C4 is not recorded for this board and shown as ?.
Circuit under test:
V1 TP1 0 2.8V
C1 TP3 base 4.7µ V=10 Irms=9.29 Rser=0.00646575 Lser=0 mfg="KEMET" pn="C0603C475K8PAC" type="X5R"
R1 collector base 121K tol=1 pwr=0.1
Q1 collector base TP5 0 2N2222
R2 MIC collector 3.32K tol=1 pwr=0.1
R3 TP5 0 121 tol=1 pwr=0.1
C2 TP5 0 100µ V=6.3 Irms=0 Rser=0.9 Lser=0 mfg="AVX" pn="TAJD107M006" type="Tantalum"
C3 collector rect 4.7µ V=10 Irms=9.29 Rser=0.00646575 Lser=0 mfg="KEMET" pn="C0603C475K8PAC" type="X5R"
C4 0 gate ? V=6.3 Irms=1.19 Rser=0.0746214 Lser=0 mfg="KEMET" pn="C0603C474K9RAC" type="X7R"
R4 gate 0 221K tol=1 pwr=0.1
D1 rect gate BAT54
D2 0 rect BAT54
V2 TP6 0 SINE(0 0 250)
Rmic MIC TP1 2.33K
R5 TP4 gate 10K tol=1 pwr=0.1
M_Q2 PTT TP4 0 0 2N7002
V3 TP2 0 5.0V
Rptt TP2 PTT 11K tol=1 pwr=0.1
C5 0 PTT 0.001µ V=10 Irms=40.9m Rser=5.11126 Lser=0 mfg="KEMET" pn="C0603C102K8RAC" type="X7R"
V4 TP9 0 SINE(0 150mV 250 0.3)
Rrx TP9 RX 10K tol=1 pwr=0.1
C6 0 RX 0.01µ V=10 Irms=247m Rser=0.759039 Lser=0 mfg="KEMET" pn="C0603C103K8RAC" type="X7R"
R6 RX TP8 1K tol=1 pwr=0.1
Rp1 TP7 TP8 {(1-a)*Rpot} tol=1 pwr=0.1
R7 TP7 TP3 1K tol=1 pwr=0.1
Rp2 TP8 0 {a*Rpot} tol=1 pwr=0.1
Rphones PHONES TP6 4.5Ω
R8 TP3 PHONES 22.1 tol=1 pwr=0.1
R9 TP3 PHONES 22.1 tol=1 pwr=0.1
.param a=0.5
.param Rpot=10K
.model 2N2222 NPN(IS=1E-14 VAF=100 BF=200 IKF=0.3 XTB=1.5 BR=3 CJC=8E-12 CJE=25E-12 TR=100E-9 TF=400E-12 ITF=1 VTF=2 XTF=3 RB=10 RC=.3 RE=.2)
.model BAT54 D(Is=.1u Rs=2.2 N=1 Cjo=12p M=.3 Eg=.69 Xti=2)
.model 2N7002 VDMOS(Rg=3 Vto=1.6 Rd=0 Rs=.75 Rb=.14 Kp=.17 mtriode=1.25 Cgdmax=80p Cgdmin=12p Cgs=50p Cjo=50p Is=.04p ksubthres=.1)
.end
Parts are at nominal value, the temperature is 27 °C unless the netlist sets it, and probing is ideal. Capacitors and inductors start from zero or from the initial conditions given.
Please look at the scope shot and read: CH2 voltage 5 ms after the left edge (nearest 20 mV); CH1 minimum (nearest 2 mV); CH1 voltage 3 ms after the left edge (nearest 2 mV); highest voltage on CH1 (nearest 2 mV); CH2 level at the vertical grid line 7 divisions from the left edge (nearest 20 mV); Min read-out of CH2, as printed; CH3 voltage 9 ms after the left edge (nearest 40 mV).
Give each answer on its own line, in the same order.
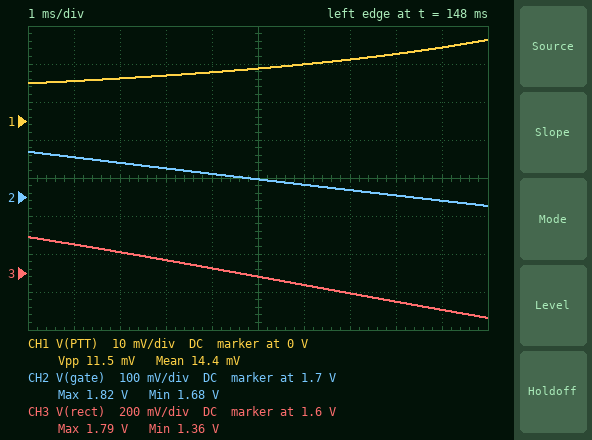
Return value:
1.74 V
10 mV
12 mV
22 mV
1.72 V
1.68 V
1.40 V
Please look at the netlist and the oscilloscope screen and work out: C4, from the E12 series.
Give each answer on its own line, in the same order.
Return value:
560 nF
